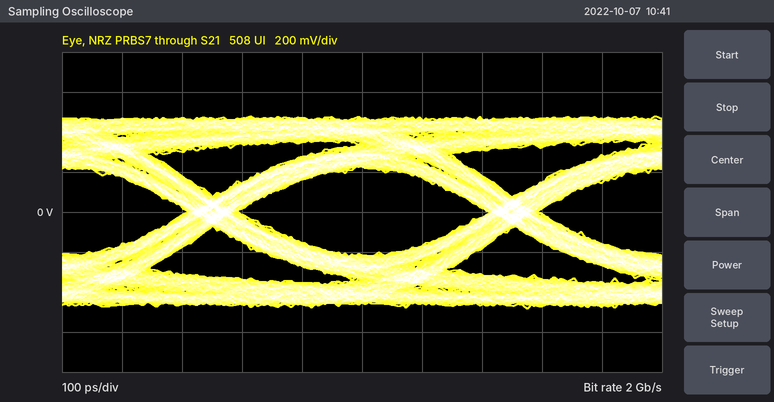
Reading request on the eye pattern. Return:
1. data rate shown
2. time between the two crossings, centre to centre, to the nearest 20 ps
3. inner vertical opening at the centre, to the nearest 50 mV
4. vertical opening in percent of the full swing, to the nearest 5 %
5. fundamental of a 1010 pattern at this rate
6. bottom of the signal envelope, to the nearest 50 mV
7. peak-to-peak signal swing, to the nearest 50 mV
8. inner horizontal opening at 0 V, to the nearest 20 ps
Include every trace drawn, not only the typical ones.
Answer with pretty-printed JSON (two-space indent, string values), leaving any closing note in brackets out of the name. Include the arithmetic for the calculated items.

{
  "data rate shown": "2 Gb/s",
  "time between the two crossings, centre to centre, to the nearest 20 ps": "500 ps",
  "inner vertical opening at the centre, to the nearest 50 mV": "450 mV",
  "vertical opening in percent of the full swing, to the nearest 5 %": "450 mV / 950 mV ≈ 47.4 %, so 45 % to the nearest 5 %",
  "fundamental of a 1010 pattern at this rate": "1 GHz",
  "bottom of the signal envelope, to the nearest 50 mV": "-500 mV",
  "peak-to-peak signal swing, to the nearest 50 mV": "950 mV",
  "inner horizontal opening at 0 V, to the nearest 20 ps": "420 ps"
}
